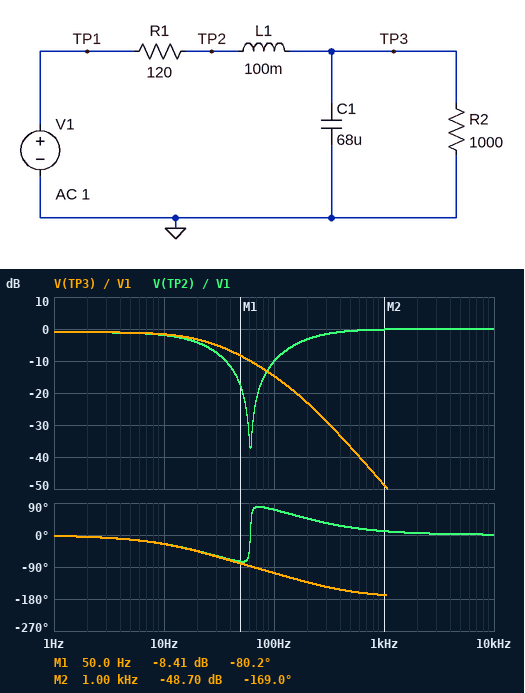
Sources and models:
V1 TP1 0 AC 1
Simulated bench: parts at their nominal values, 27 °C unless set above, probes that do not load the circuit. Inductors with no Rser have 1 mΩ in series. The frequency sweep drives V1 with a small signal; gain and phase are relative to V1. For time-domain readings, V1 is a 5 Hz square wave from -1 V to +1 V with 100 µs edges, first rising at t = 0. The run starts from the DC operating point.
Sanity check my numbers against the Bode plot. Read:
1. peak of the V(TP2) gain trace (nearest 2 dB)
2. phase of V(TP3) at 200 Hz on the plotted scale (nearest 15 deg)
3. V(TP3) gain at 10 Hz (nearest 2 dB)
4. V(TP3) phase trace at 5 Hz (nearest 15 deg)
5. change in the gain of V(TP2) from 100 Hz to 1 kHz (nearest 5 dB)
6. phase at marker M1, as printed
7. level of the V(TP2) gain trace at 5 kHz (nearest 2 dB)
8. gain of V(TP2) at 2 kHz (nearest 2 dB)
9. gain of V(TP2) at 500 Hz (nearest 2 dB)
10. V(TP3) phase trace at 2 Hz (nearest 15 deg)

0 dB
-135 deg
-2 dB
-15 deg
10 dB
-80.2 deg
0 dB
0 dB
0 dB
0 deg
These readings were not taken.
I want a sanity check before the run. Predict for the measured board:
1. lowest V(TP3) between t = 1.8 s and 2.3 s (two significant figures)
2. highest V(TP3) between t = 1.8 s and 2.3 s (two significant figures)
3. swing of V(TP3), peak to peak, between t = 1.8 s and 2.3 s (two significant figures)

-890 mV
890 mV
1.8 V
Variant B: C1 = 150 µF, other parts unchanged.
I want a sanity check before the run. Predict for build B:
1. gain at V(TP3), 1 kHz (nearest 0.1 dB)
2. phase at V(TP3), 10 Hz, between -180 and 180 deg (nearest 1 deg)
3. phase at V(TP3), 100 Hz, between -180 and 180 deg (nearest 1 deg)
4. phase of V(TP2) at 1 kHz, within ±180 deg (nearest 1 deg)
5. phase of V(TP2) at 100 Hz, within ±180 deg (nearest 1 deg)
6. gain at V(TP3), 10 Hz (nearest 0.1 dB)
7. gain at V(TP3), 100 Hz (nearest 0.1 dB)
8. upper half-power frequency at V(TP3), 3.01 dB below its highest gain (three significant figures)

-55.6 dB
-47 deg
-113 deg
11 deg
66 deg
-3.8 dB
-21.8 dB
10.4 Hz
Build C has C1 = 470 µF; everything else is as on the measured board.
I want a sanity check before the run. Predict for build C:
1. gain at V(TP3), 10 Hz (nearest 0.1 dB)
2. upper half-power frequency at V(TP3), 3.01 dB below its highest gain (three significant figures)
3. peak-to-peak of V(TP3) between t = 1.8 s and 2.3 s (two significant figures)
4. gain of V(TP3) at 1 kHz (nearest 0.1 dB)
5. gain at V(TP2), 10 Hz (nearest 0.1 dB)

-11.3 dB
3.21 Hz
1.4 V
-65.5 dB
-13.1 dB
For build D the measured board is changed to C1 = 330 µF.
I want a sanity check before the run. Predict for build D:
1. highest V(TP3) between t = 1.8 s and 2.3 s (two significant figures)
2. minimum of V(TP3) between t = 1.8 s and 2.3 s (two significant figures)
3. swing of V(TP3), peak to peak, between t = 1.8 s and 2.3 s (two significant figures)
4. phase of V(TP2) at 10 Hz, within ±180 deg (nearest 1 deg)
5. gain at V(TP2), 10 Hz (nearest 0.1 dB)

800 mV
-800 mV
1.6 V
-68 deg
-9.8 dB
